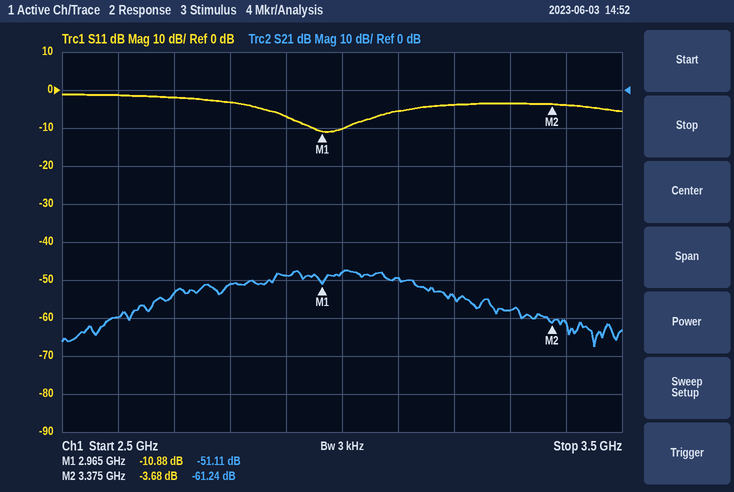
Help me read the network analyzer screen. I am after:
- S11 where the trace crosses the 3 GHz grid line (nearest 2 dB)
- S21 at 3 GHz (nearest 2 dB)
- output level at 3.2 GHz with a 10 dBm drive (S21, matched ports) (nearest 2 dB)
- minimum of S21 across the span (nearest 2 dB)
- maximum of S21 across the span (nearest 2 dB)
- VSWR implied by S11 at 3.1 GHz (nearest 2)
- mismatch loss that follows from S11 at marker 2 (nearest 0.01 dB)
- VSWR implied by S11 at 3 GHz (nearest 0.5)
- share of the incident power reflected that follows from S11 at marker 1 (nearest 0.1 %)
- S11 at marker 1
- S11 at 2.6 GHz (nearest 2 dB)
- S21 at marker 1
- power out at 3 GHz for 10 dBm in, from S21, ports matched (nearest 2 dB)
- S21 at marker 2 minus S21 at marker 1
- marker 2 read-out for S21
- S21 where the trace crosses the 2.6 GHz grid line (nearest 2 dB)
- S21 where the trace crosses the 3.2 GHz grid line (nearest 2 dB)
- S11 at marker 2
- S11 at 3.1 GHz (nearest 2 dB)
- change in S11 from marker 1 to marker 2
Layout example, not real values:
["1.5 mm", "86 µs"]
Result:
["-10 dB", "-48 dB", "-44 dBm", "-68 dB", "-48 dB", "4", "2.43 dB", "2.0", "8.2 %", "-10.88 dB", "-2 dB", "-51.11 dB", "-38 dBm", "-10.13 dB", "-61.24 dB", "-60 dB", "-54 dB", "-3.68 dB", "-6 dB", "7.20 dB"]
